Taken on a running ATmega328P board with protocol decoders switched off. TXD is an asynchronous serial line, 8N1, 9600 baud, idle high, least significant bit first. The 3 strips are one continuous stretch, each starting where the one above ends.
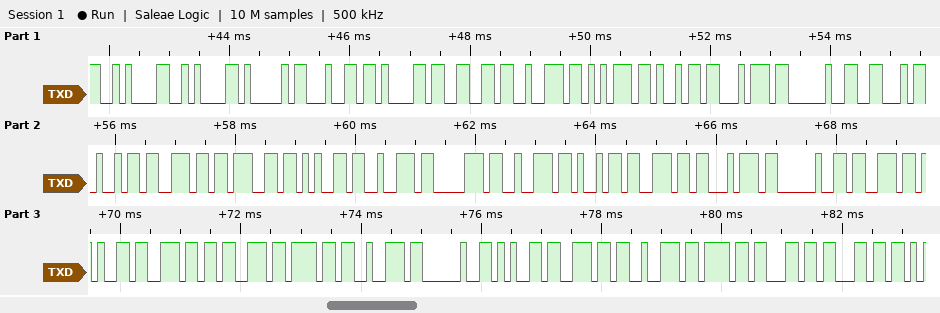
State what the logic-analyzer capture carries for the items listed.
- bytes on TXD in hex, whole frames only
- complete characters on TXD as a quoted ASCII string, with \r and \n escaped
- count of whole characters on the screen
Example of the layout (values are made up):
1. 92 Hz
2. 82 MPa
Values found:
1. 0A 0A 41 64 61 66 72 75 69 74 20 46 69 6E 67 65 72 70 72 69 6E 74 20 73 65 6E 73 6F 72 20 65 6E 72 6F 6C 6C
2. "\n\nAdafruit Fingerprint sensor enroll"
3. 36
